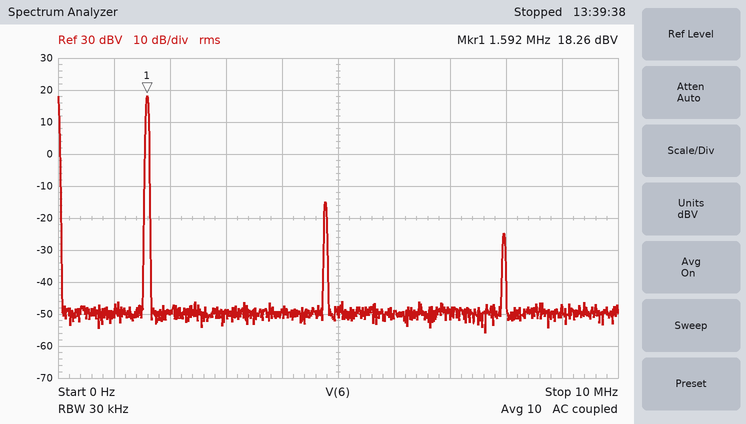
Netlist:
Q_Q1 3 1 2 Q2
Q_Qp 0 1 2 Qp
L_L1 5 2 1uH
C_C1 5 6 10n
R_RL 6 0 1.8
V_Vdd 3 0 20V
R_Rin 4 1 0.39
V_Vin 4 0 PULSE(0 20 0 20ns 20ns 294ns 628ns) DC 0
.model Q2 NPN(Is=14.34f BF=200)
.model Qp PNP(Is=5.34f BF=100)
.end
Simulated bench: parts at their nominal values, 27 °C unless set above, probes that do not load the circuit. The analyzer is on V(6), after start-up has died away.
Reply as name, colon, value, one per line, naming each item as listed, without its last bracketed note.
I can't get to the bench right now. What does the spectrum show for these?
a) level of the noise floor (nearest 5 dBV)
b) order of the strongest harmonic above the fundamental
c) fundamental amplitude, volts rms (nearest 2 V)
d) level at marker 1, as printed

level of the noise floor: -50 dBV
order of the strongest harmonic above the fundamental: 3
fundamental amplitude, volts rms: 8 V
level at marker 1, as printed: 18.26 dBV
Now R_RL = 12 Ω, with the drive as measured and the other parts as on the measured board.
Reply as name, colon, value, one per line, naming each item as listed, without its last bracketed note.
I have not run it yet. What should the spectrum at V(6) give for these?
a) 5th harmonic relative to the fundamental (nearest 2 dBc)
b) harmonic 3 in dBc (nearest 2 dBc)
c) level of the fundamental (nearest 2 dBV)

5th harmonic relative to the fundamental: -26 dBc
harmonic 3 in dBc: -18 dBc
level of the fundamental: 18 dBV
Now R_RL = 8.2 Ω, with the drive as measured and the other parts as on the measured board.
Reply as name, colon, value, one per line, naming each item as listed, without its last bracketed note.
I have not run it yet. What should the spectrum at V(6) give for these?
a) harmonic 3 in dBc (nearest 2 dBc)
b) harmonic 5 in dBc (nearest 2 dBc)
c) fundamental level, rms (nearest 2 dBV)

harmonic 3 in dBc: -20 dBc
harmonic 5 in dBc: -30 dBc
fundamental level, rms: 18 dBV
